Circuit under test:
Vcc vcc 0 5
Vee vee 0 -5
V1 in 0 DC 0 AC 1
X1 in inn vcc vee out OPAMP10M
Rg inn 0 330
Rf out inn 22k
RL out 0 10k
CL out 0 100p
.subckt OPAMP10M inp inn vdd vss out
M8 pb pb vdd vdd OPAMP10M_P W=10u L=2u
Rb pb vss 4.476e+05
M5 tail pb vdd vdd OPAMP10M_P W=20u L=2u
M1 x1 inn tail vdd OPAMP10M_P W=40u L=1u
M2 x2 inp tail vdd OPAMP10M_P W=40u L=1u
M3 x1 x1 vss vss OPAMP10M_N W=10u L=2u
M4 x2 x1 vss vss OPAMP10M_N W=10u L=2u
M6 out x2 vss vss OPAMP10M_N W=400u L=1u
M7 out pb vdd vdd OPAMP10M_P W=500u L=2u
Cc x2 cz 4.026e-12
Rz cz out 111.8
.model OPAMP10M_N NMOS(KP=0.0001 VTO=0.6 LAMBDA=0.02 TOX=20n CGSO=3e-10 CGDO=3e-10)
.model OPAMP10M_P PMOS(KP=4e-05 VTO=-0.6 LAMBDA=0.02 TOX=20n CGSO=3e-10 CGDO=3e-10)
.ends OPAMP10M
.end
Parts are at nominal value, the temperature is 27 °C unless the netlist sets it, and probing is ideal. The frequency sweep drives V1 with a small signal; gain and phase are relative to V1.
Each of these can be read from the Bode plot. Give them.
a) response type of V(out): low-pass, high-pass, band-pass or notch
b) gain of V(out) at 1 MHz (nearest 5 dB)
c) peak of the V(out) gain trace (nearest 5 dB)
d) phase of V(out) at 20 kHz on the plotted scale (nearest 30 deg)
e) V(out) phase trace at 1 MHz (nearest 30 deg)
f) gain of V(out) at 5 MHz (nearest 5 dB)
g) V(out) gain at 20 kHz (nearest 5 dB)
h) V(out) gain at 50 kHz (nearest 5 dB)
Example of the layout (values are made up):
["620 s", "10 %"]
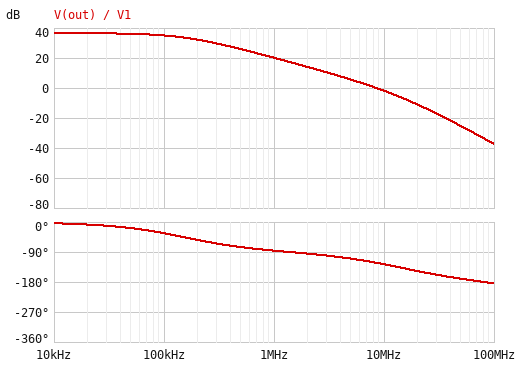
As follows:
["low-pass", "20 dB", "35 dB", "0 deg", "-90 deg", "5 dB", "35 dB", "35 dB"]
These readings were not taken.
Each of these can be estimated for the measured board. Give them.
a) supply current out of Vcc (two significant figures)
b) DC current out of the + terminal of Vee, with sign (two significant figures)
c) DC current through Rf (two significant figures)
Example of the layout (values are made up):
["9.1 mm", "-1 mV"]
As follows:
["1.1 mA", "-1.1 mA", "600 nA"]
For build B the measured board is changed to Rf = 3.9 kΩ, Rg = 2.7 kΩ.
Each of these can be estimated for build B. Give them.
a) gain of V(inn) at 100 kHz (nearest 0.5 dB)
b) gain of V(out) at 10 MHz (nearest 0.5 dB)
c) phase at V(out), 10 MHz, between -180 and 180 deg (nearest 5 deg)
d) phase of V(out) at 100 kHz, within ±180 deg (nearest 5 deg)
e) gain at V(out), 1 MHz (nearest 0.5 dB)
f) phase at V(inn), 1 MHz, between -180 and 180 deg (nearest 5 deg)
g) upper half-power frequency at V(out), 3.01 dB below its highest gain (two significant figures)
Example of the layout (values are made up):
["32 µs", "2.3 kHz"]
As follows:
["0 dB", "-0.5 dB", "-110 deg", "0 deg", "7.5 dB", "-15 deg", "5.5 MHz"]
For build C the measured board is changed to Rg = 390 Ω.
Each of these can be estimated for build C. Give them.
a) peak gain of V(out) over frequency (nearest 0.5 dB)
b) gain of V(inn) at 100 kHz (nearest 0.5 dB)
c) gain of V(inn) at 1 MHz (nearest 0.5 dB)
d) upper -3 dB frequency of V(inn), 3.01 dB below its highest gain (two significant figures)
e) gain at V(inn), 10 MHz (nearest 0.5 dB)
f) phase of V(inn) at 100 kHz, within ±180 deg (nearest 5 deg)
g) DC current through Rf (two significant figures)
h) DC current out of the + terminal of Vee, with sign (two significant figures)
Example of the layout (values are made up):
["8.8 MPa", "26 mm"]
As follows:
["35.0 dB", "-1.0 dB", "-15.0 dB", "180 kHz", "-37.5 dB", "-30 deg", "510 nA", "-1.1 mA"]
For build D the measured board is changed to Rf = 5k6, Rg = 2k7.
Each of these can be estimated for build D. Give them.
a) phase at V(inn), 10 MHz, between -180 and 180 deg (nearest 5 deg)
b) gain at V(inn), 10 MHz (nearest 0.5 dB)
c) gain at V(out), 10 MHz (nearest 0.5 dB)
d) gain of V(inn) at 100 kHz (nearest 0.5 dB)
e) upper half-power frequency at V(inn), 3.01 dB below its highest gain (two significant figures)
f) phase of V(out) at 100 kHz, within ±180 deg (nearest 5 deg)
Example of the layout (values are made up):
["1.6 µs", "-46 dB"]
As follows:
["-115 deg", "-10.5 dB", "-0.5 dB", "0 dB", "4.2 MHz", "0 deg"]
